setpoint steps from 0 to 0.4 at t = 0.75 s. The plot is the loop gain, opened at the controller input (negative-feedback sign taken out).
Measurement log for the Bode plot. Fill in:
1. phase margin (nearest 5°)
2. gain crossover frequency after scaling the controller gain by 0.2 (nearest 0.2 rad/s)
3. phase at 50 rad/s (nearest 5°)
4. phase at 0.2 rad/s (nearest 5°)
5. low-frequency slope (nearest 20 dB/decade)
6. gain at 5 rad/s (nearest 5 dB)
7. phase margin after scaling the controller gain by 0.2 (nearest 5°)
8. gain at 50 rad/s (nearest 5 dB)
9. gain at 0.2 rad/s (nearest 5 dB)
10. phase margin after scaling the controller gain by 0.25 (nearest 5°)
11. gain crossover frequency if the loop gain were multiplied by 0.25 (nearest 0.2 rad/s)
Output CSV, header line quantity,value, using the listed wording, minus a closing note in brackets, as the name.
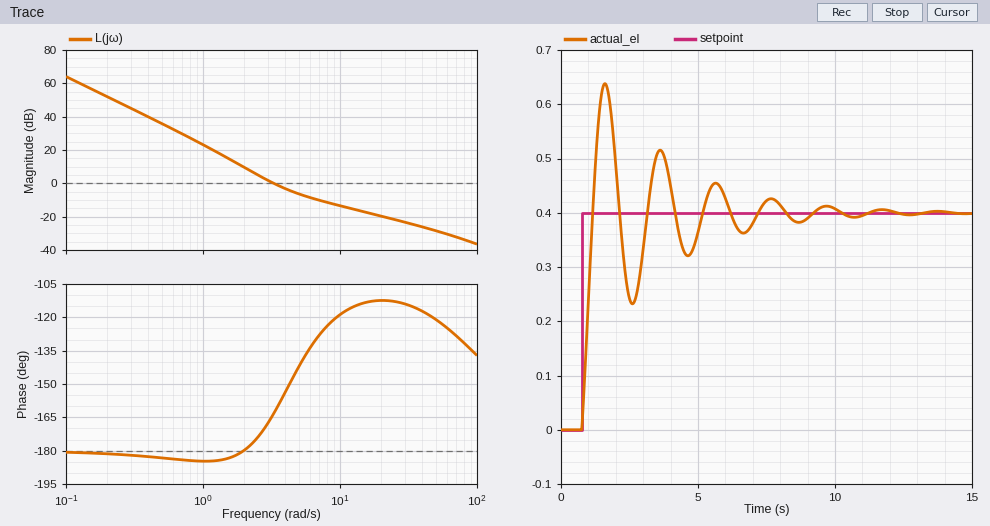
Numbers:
quantity,value
phase margin,15°
gain crossover frequency after scaling the controller gain by 0.2,1.6 rad/s
phase at 50 rad/s,-120°
phase at 0.2 rad/s,-180°
low-frequency slope,-40 dB/decade
gain at 5 rad/s,-5 dB
phase margin after scaling the controller gain by 0.2,-5°
gain at 50 rad/s,-30 dB
gain at 0.2 rad/s,50 dB
phase margin after scaling the controller gain by 0.25,0°
gain crossover frequency if the loop gain were multiplied by 0.25,1.8 rad/s
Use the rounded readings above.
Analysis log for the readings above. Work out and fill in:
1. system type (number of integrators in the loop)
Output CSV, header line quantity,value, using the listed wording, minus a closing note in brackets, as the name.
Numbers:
quantity,value
system type,2
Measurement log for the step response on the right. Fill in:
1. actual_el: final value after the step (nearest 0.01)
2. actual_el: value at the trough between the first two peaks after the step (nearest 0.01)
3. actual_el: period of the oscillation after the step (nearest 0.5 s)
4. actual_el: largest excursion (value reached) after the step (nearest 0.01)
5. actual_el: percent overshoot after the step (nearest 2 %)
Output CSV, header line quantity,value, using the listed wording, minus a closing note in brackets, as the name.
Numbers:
quantity,value
actual_el: final value after the step,0.40
actual_el: value at the trough between the first two peaks after the step,0.23
actual_el: period of the oscillation after the step,2.0 s
actual_el: largest excursion (value reached) after the step,0.64
actual_el: percent overshoot after the step,60 %
